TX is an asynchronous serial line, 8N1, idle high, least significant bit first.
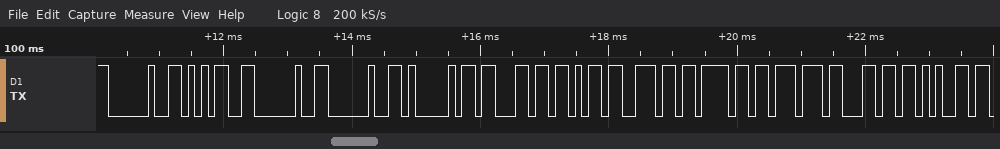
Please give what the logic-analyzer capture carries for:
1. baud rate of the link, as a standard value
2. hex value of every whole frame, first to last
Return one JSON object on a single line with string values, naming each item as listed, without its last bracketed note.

{"baud rate of the link, as a standard value": "9600 baud", "hex value of every whole frame, first to last": "0x20 0x35 0x20 0x20 0x41 0x63 0x6B 0x6E 0x6F 0x77 0x6C 0x65"}
